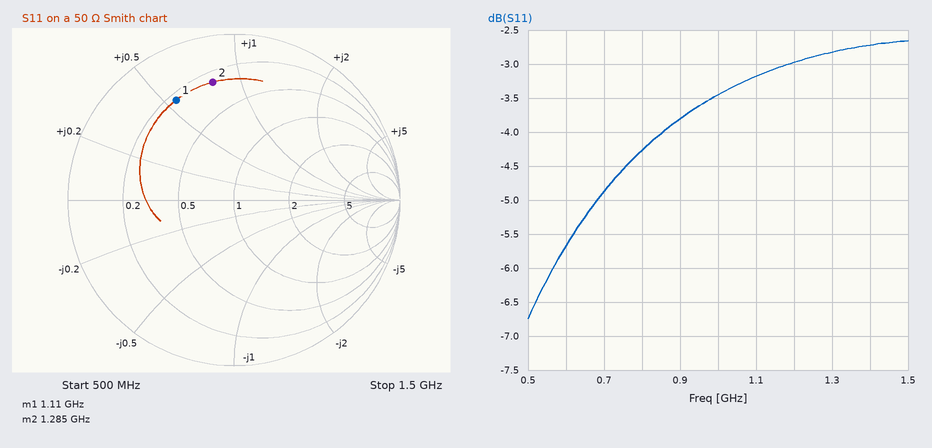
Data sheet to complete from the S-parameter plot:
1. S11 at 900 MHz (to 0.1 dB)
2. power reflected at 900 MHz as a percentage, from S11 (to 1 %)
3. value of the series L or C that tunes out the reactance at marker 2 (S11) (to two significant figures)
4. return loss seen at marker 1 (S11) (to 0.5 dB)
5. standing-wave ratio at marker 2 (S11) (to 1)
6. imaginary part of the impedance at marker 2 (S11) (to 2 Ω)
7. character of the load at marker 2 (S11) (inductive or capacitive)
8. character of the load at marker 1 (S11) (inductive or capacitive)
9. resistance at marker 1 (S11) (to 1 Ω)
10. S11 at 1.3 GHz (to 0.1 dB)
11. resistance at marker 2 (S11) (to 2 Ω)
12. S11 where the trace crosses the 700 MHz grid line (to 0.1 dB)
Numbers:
-3.8 dB
42 %
3.1 pF
3.0 dB
6
+40 Ω
inductive
inductive
12 Ω
-2.8 dB
14 Ω
-4.9 dB
